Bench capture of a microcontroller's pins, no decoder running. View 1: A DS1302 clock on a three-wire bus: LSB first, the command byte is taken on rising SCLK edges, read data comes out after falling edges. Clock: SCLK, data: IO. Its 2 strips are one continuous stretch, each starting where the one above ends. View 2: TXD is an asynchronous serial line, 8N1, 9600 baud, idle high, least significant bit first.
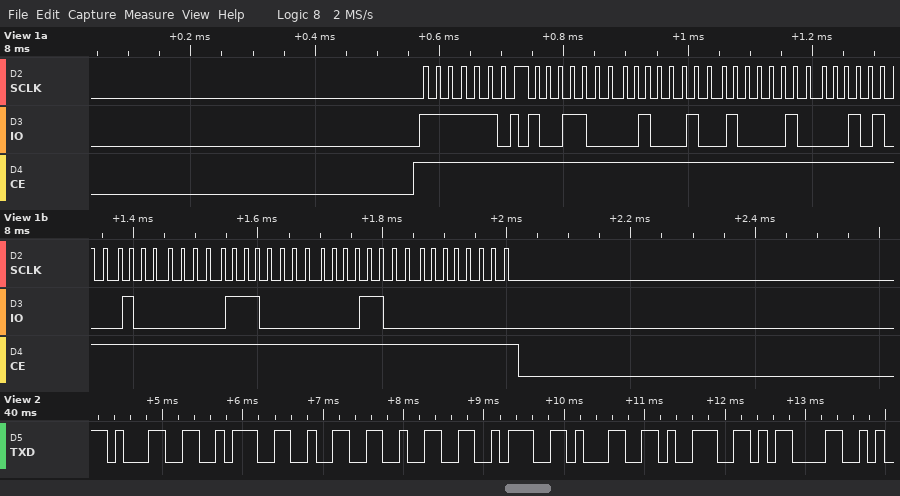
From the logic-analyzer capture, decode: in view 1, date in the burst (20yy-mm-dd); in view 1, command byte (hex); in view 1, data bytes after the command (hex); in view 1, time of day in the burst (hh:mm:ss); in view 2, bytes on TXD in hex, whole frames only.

2018-01-14
0xBF
19 22 21 14 01 07 18 00
21:22:19
31 3A 32 32 3A 31 39 0D
